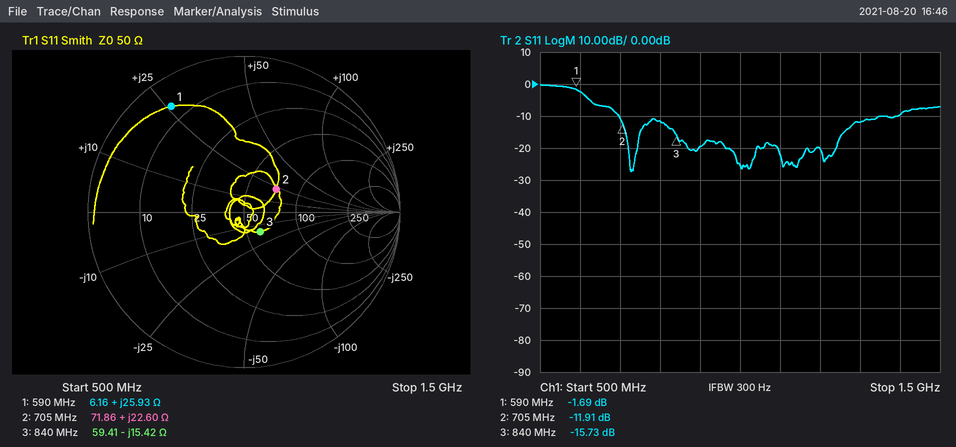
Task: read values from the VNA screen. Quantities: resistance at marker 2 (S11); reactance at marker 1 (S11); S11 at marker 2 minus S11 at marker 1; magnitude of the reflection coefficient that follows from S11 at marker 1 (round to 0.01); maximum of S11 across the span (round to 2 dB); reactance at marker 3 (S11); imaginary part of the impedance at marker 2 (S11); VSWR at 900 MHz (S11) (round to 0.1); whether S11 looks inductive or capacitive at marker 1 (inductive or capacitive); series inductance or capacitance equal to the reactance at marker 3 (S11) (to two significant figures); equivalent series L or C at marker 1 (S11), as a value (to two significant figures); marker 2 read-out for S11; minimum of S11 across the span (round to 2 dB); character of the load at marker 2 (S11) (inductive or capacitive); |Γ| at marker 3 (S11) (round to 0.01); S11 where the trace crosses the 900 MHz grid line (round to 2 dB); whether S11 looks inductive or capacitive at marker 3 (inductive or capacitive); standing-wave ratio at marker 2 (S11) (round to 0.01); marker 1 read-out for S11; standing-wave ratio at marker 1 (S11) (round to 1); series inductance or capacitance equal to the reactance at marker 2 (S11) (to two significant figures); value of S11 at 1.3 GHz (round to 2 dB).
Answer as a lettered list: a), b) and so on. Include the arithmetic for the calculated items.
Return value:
a) 71.86 Ω
b) +25.93 Ω
c) -11.91 − (-1.69) = -10.22 dB
d) 10^(-1.69/20) ≈ 0.82
e) 0 dB
f) -15.42 Ω
g) +22.60 Ω
h) |Γ| = 10^(-20/20) = 0.1000; VSWR = (1 + 0.1000)/(1 − 0.1000) ≈ 1.2
i) inductive
j) C = 1/(2π × 840 MHz × 15.42 Ω) ≈ 12 pF
k) L = 25.93 Ω/(2π × 590 MHz) ≈ 7.0 nH
l) -11.91 dB
m) -28 dB
n) inductive
o) 0.16
p) -20 dB
q) capacitive
r) 1.68
s) -1.69 dB
t) 10
u) L = 22.6 Ω/(2π × 705 MHz) ≈ 5.1 nH
v) -12 dB
